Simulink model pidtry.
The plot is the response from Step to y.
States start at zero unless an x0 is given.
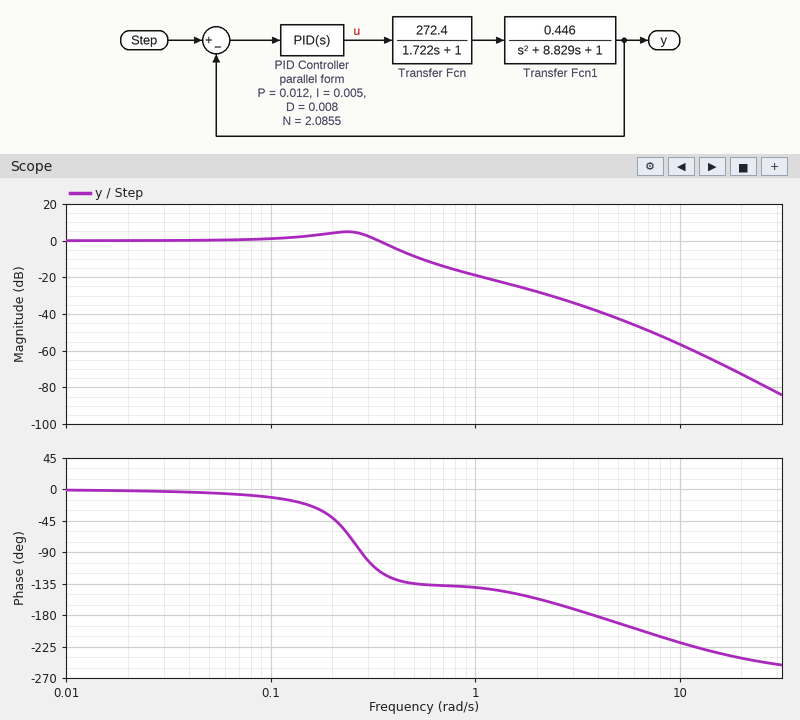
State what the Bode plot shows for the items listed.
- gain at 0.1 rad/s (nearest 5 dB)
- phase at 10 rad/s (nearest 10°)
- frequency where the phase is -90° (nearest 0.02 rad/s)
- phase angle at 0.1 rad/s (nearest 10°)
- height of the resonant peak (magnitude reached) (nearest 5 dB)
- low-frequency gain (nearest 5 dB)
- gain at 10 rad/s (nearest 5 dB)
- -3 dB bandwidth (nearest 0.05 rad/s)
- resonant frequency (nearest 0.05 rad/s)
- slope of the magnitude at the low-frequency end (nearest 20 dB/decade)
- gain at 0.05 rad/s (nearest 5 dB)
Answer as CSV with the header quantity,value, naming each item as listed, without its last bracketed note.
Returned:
quantity,value
gain at 0.1 rad/s,0 dB
phase at 10 rad/s,-220°
frequency where the phase is -90°,0.28 rad/s
phase angle at 0.1 rad/s,-10°
height of the resonant peak (magnitude reached),5 dB
low-frequency gain,0 dB
gain at 10 rad/s,-55 dB
-3 dB bandwidth,0.40 rad/s
resonant frequency,0.25 rad/s
slope of the magnitude at the low-frequency end,0 dB/decade
gain at 0.05 rad/s,0 dB
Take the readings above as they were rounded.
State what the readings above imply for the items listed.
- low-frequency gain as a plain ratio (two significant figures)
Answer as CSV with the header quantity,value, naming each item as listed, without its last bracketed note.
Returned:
quantity,value
low-frequency gain as a plain ratio,1.0
